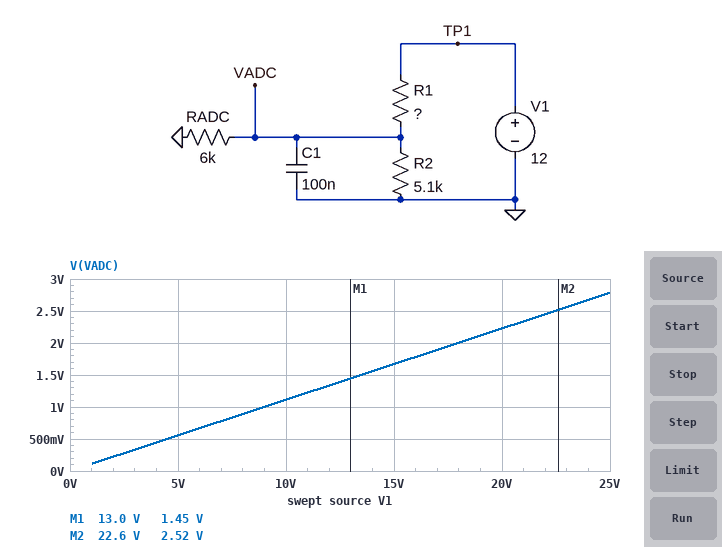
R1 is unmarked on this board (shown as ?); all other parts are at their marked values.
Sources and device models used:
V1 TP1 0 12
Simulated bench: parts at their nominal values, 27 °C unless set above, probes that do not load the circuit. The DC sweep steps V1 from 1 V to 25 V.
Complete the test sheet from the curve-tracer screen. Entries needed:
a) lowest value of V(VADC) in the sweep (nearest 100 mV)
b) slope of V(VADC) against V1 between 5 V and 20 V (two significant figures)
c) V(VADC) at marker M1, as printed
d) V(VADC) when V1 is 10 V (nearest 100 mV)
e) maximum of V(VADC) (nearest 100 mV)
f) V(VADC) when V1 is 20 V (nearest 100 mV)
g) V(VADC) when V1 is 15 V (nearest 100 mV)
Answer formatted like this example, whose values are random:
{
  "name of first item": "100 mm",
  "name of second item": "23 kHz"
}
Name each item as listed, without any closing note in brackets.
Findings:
{
  "lowest value of V(VADC) in the sweep": "100 mV",
  "slope of V(VADC) against V1 between 5 V and 20 V": "0.11 V/V",
  "V(VADC) at marker M1, as printed": "1.45 V",
  "V(VADC) when V1 is 10 V": "1.1 V",
  "maximum of V(VADC)": "2.8 V",
  "V(VADC) when V1 is 20 V": "2.2 V",
  "V(VADC) when V1 is 15 V": "1.7 V"
}
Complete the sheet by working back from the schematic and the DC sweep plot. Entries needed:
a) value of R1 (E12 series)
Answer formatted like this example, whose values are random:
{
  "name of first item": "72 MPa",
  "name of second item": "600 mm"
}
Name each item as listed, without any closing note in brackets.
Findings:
{
  "value of R1": "22 kΩ"
}
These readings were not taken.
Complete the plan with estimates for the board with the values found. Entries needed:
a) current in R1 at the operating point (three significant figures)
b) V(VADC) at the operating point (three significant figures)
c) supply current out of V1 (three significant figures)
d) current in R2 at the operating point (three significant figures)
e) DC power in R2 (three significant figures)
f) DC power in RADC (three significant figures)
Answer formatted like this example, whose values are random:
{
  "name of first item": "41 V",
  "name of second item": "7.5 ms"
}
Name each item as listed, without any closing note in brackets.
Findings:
{
  "current in R1 at the operating point": "485 µA",
  "V(VADC) at the operating point": "1.34 V",
  "supply current out of V1": "485 µA",
  "current in R2 at the operating point": "262 µA",
  "DC power in R2": "350 µW",
  "DC power in RADC": "298 µW"
}
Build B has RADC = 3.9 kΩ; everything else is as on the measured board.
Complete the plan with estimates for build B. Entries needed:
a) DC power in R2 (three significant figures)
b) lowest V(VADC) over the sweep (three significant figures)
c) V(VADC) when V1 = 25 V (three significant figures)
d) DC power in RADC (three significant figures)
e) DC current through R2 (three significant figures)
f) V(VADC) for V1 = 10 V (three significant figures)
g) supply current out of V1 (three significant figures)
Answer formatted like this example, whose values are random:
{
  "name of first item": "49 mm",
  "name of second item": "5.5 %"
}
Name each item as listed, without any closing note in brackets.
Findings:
{
  "DC power in R2": "235 µW",
  "lowest V(VADC) over the sweep": "91.3 mV",
  "V(VADC) when V1 = 25 V": "2.28 V",
  "DC power in RADC": "308 µW",
  "DC current through R2": "215 µA",
  "V(VADC) for V1 = 10 V": "913 mV",
  "supply current out of V1": "496 µA"
}
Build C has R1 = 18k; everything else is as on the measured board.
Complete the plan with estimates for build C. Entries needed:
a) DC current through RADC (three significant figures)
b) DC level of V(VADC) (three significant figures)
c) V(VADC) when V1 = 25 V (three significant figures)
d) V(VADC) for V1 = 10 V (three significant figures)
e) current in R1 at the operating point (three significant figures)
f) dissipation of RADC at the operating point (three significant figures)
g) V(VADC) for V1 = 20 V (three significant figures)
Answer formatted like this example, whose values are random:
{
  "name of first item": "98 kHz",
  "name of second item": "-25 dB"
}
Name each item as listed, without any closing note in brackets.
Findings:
{
  "DC current through RADC": "266 µA",
  "DC level of V(VADC)": "1.59 V",
  "V(VADC) when V1 = 25 V": "3.32 V",
  "V(VADC) for V1 = 10 V": "1.33 V",
  "current in R1 at the operating point": "578 µA",
  "dissipation of RADC at the operating point": "423 µW",
  "V(VADC) for V1 = 20 V": "2.66 V"
}
